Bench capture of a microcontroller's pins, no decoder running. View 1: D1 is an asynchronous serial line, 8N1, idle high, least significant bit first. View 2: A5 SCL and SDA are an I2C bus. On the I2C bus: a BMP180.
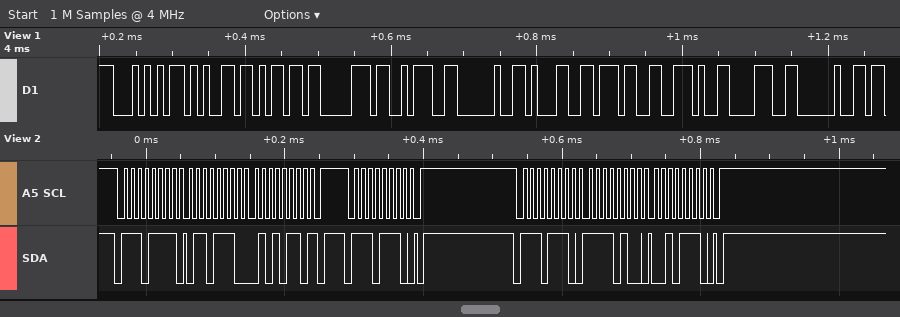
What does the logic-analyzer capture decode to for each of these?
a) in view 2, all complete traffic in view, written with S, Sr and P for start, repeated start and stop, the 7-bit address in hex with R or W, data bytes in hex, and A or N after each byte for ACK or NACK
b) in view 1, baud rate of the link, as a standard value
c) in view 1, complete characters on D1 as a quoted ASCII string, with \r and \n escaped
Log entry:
S 77R A 6E A 56 N P S 77W A P S 77W A F4 A 2E A P
115200 baud
"Temp: 17.8 "
